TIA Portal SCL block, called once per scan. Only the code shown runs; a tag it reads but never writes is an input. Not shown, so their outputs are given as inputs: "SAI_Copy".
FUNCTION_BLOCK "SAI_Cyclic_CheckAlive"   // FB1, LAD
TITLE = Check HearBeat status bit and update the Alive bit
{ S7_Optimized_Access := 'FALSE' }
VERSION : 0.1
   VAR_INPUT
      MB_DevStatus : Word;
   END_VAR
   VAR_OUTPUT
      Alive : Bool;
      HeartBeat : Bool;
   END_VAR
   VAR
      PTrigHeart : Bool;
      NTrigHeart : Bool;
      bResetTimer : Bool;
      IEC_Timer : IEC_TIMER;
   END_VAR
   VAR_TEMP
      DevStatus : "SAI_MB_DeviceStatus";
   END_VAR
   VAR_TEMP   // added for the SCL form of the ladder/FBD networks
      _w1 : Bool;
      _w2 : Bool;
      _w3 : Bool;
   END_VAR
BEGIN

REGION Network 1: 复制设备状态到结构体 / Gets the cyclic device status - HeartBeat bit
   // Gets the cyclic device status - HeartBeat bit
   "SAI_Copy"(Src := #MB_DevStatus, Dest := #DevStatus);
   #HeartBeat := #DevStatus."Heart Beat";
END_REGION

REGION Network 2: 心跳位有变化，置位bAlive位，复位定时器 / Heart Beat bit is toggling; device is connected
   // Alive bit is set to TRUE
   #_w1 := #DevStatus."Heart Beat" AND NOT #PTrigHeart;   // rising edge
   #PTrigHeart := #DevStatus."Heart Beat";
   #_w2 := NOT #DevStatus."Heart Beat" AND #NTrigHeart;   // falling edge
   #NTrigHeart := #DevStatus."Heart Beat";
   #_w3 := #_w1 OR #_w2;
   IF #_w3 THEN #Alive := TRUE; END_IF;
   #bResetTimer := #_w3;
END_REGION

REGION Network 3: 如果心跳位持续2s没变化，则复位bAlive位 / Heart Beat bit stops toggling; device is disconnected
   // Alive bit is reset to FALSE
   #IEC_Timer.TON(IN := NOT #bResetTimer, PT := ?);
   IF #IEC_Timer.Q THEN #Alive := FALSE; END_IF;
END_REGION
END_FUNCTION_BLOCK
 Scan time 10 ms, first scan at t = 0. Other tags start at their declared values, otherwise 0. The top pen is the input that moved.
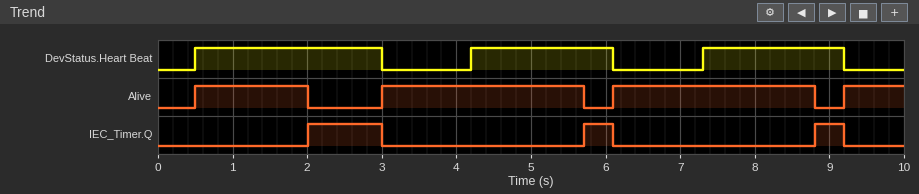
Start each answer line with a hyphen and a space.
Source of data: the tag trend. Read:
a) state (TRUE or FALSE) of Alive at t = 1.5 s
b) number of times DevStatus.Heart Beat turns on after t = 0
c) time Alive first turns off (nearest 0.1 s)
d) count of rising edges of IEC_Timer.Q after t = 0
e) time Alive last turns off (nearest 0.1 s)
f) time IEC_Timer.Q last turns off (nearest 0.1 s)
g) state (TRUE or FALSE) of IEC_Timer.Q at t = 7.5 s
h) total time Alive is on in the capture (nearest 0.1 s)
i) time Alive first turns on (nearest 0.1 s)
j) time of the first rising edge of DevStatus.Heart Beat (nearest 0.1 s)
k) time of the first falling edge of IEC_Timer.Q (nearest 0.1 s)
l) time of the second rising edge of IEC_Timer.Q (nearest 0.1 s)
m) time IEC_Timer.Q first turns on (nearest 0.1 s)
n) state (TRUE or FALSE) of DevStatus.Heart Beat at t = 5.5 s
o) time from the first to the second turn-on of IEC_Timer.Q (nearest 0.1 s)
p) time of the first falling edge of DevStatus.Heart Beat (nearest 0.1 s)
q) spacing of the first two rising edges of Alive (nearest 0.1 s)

- TRUE
- 3
- 2.0 s
- 3
- 8.8 s
- 9.2 s
- FALSE
- 7.7 s
- 0.5 s
- 0.5 s
- 3.0 s
- 5.7 s
- 2.0 s
- TRUE
- 3.7 s
- 3.0 s
- 2.5 s
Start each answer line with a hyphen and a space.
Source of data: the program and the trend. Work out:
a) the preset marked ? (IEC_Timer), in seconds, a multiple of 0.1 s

- 1.5 s
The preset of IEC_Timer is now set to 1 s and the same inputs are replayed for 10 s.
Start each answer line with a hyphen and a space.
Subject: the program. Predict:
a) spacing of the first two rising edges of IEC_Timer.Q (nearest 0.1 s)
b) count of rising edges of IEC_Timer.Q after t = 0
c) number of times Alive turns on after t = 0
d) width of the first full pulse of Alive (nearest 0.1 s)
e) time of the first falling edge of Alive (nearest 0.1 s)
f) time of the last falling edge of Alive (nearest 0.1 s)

- 2.5 s
- 5
- 6
- 1.0 s
- 1.5 s
- 8.3 s
